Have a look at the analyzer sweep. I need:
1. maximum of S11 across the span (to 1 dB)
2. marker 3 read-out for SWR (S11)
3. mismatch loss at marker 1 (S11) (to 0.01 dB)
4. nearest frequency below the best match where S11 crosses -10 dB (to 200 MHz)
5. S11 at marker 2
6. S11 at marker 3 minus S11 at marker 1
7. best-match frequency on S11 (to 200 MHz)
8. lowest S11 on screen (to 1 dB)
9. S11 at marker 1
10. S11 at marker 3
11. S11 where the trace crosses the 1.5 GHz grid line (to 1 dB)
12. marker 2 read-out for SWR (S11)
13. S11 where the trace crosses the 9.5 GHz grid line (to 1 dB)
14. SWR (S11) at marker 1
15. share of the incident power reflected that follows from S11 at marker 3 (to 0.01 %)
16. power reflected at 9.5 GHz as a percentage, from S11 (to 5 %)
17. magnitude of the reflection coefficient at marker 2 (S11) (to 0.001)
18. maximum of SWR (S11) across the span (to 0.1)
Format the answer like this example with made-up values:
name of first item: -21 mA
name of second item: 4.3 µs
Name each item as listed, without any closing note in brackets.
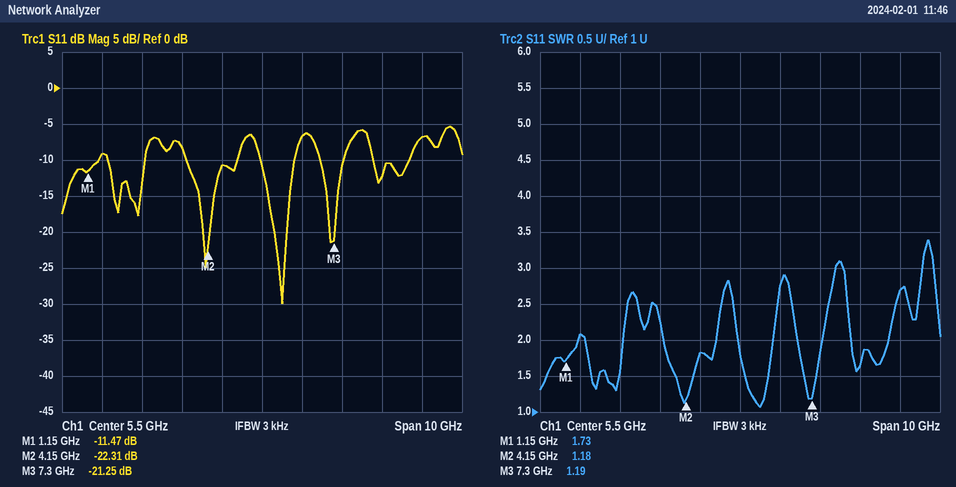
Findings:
maximum of S11 across the span: -5 dB
marker 3 read-out for SWR: 1.19
mismatch loss at marker 1 (S11): 0.32 dB
nearest frequency below the best match where S11 crosses -10 dB: 5.4 GHz
S11 at marker 2: -22.31 dB
S11 at marker 3 minus S11 at marker 1: -9.78 dB
best-match frequency on S11: 6.0 GHz
lowest S11 on screen: -30 dB
S11 at marker 1: -11.47 dB
S11 at marker 3: -21.25 dB
S11 where the trace crosses the 1.5 GHz grid line: -9 dB
marker 2 read-out for SWR: 1.18
S11 where the trace crosses the 9.5 GHz grid line: -7 dB
SWR (S11) at marker 1: 1.73
share of the incident power reflected that follows from S11 at marker 3: 0.75 %
power reflected at 9.5 GHz as a percentage, from S11: 20 %
magnitude of the reflection coefficient at marker 2 (S11): 0.077
maximum of SWR (S11) across the span: 3.4
